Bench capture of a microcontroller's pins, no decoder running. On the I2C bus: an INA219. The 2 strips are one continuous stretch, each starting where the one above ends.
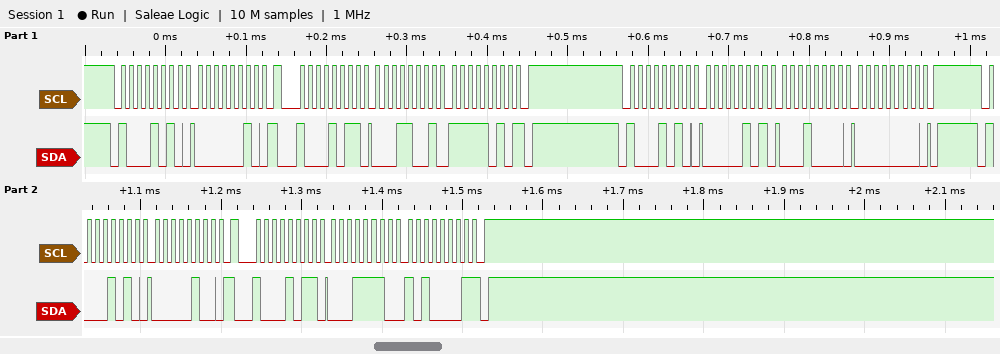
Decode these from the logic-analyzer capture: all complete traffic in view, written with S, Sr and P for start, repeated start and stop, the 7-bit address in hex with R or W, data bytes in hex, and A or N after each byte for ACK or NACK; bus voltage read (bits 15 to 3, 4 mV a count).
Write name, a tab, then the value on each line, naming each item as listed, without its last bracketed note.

all complete traffic in view, written with S, Sr and P for start, repeated start and stop, the 7-bit address in hex with R or W, data bytes in hex, and A or N after each byte for ACK or NACK	S 45W A 02 A Sr 45R A 19 A FA N P S 45W A 05 A 10 A 00 A P S 45W A 04 A Sr 45R A 1E A A1 N P
bus voltage read	3.324 V
